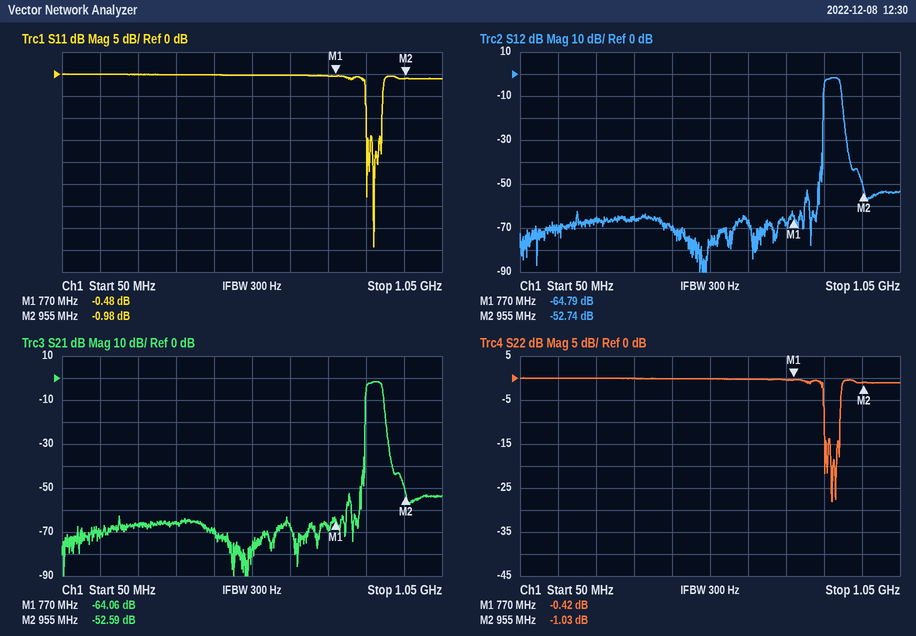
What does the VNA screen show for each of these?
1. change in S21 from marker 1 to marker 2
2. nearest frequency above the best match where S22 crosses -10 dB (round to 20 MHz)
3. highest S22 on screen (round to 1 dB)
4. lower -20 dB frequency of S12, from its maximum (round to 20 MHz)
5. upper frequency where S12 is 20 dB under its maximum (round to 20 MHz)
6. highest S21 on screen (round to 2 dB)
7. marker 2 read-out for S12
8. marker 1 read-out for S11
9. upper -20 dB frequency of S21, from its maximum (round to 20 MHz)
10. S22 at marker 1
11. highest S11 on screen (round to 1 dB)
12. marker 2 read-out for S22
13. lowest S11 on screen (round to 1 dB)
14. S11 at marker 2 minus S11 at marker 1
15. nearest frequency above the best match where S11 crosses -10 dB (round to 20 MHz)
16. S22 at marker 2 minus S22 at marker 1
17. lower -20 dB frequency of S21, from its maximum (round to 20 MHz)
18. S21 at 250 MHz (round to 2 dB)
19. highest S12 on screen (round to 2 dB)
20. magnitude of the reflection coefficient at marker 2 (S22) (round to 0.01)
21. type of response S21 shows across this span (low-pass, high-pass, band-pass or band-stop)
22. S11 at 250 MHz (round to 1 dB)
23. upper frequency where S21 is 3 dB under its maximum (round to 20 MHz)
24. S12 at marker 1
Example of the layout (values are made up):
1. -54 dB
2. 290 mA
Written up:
1. 11.47 dB
2. 900 MHz
3. 0 dB
4. 840 MHz
5. 900 MHz
6. -2 dB
7. -52.74 dB
8. -0.48 dB
9. 900 MHz
10. -0.42 dB
11. 0 dB
12. -1.03 dB
13. -39 dB
14. -0.50 dB
15. 900 MHz
16. -0.61 dB
17. 840 MHz
18. -66 dB
19. -2 dB
20. 0.89
21. band-pass
22. 0 dB
23. 900 MHz
24. -64.79 dB
